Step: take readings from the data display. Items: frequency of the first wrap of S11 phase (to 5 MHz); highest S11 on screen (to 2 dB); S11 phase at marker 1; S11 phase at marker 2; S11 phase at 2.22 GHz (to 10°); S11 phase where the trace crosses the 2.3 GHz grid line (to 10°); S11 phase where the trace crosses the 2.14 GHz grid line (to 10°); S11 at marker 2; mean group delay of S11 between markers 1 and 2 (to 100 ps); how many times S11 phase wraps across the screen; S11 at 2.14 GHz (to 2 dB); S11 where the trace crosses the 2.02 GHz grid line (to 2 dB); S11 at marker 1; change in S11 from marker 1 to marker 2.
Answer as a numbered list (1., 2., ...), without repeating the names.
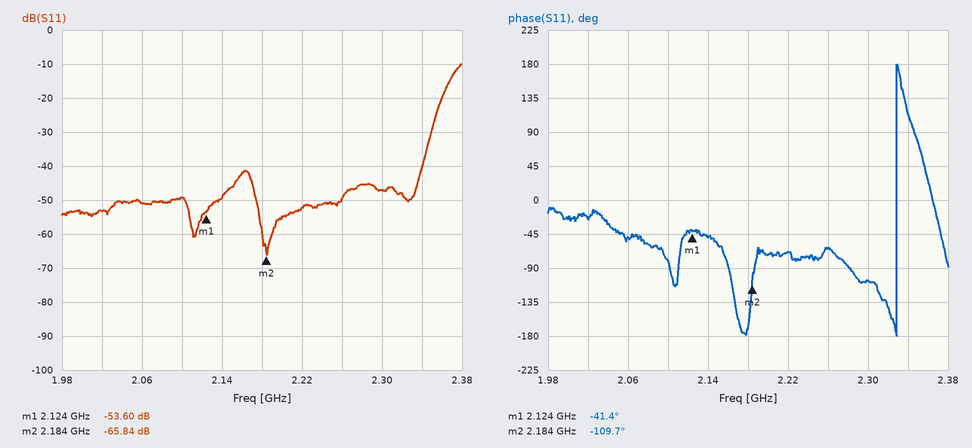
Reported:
1. 2.330 GHz
2. -10 dB
3. -41.4°
4. -109.7°
5. -70°
6. -110°
7. -50°
8. -65.84 dB
9. 3.2 ns
10. 1
11. -50 dB
12. -54 dB
13. -53.60 dB
14. -12.24 dB
